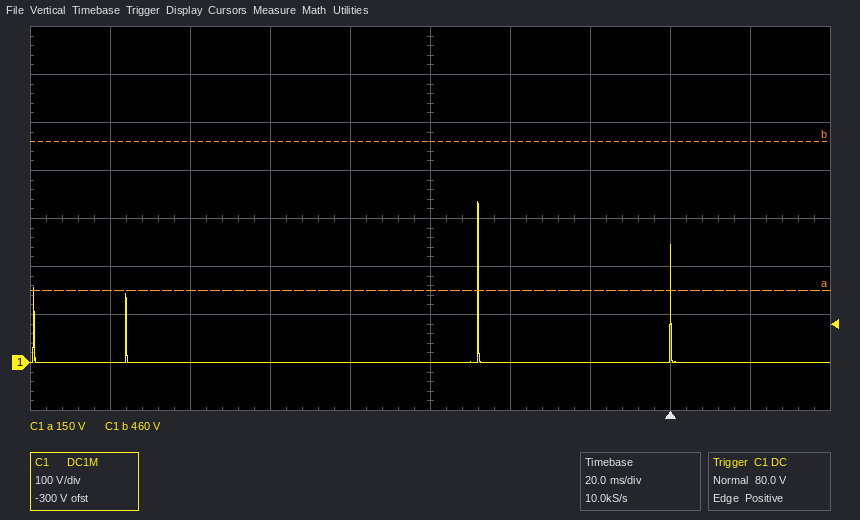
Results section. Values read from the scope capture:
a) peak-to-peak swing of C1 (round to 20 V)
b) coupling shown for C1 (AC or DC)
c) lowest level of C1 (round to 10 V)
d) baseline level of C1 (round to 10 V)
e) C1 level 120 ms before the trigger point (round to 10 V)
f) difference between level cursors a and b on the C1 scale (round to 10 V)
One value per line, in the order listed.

340 V
DC
0 V
0 V
0 V
310 V
